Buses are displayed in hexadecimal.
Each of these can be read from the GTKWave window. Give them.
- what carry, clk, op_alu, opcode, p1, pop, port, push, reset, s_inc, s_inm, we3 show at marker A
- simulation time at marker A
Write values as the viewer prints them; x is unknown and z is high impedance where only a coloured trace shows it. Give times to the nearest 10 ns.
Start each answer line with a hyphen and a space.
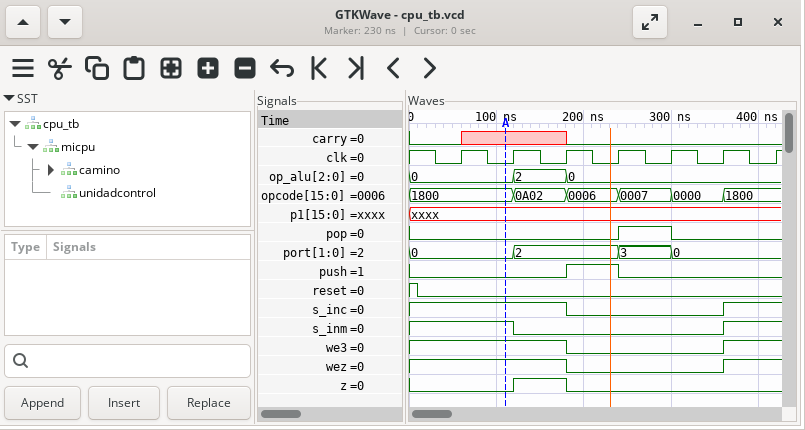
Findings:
- carry=x, clk=0, op_alu=0, opcode=1800, p1=xxxx, pop=0, port=0, push=0, reset=0, s_inc=1, s_inm=1, we3=1
- 110 ns
